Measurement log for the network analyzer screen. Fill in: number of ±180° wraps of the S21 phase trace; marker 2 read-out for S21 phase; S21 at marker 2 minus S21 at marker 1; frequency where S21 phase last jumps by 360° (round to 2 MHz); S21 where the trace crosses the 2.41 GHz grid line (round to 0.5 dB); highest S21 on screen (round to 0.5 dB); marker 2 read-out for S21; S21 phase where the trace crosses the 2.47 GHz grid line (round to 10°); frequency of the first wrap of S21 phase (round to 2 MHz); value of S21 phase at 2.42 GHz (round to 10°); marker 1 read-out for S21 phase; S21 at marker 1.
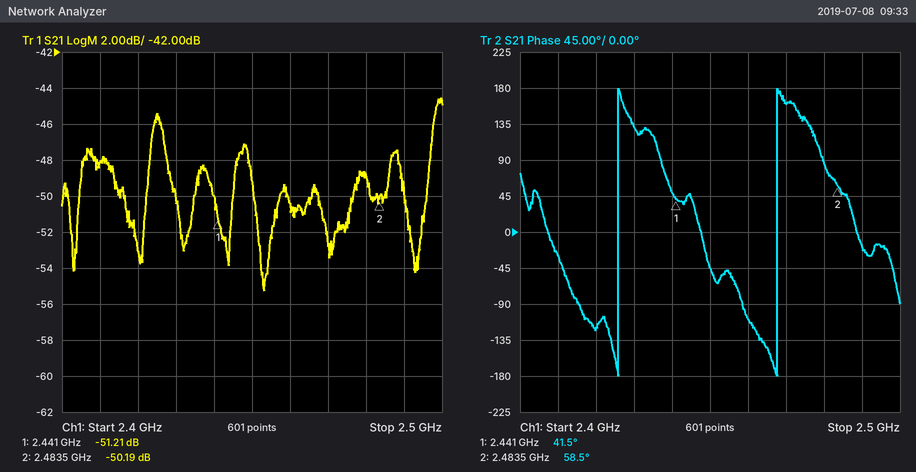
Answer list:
2
58.5°
1.02 dB
2.468 GHz
-48.0 dB
-44.5 dB
-50.19 dB
160°
2.426 GHz
-120°
41.5°
-51.21 dB
